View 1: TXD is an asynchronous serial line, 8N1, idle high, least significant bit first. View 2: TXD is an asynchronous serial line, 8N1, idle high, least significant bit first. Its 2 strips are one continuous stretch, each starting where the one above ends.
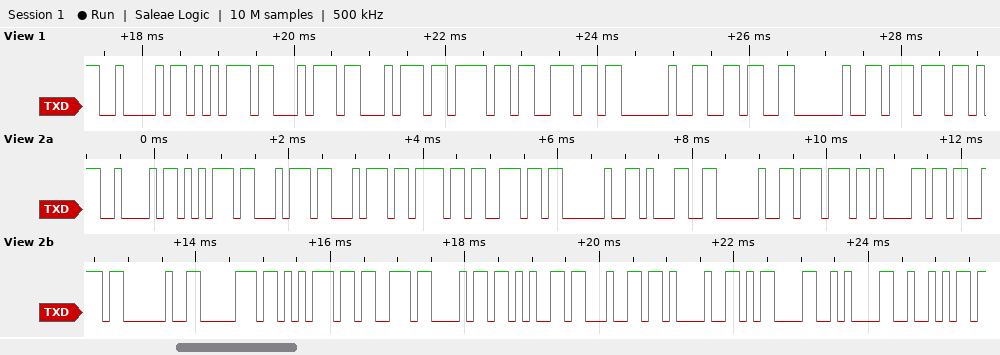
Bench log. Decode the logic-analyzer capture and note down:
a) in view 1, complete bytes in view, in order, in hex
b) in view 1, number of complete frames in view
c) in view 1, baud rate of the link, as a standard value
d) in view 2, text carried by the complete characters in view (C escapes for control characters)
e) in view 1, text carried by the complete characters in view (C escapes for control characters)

42 75 74 74 6F 6E 20 36 20 77
10
9600 baud
"Button 1 was pushed!\r\nR"
"Button 6 w"
